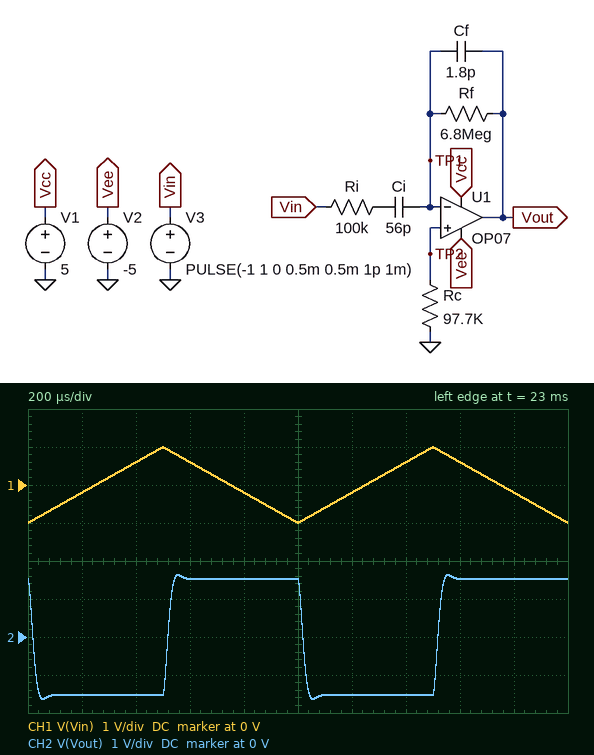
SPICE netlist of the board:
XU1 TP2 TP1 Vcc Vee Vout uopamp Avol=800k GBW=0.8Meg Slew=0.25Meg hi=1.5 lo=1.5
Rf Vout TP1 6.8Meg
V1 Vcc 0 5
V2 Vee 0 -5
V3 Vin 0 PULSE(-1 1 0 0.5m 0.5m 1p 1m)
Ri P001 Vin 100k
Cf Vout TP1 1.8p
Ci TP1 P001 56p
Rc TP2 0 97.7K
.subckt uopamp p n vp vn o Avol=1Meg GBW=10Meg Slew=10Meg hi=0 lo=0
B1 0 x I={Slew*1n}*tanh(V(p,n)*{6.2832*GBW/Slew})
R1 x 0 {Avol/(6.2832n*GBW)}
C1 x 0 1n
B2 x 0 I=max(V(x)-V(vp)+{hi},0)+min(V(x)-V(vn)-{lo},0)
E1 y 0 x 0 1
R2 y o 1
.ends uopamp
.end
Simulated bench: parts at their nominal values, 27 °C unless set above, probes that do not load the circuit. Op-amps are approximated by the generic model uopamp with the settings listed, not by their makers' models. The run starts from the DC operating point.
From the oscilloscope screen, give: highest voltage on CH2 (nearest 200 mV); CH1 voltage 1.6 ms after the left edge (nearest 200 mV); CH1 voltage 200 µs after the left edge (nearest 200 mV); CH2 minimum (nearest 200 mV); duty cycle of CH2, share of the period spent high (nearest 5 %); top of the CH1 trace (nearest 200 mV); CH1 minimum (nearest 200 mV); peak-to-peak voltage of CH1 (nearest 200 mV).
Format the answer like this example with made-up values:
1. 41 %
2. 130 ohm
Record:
1. 1.6 V
2. 600 mV
3. -200 mV
4. -1.6 V
5. 50 %
6. 1.0 V
7. -1.0 V
8. 2.0 V
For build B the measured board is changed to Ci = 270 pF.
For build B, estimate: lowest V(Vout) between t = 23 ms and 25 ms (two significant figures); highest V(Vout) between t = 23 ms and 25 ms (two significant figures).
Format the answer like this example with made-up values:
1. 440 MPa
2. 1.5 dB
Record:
1. -3.5 V
2. 3.5 V
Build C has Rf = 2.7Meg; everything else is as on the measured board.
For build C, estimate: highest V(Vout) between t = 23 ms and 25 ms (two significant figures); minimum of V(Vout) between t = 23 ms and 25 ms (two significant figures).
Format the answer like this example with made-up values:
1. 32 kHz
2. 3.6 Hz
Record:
1. 670 mV
2. -670 mV
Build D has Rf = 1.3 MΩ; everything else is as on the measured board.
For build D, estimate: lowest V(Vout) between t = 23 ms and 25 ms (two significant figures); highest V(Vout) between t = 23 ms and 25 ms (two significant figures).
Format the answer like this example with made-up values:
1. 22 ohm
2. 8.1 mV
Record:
1. -310 mV
2. 310 mV
